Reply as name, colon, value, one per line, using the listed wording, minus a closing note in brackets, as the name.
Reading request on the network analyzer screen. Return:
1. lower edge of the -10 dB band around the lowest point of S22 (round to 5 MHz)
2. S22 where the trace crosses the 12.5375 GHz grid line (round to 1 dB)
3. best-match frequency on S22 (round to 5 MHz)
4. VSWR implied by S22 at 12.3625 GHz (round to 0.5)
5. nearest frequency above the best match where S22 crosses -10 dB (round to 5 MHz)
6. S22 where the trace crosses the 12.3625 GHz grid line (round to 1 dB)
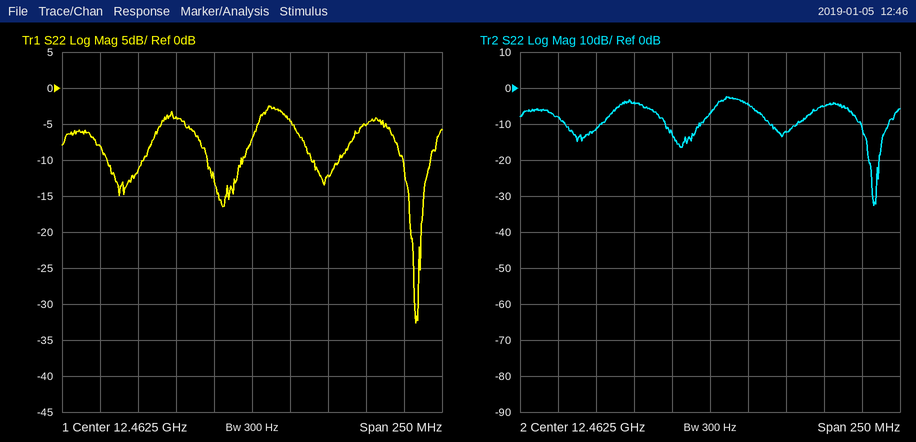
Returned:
lower edge of the -10 dB band around the lowest point of S22: 12.560 GHz
S22 where the trace crosses the 12.5375 GHz grid line: -5 dB
best-match frequency on S22: 12.570 GHz
VSWR implied by S22 at 12.3625 GHz: 2.5
nearest frequency above the best match where S22 crosses -10 dB: 12.580 GHz
S22 where the trace crosses the 12.3625 GHz grid line: -8 dB
